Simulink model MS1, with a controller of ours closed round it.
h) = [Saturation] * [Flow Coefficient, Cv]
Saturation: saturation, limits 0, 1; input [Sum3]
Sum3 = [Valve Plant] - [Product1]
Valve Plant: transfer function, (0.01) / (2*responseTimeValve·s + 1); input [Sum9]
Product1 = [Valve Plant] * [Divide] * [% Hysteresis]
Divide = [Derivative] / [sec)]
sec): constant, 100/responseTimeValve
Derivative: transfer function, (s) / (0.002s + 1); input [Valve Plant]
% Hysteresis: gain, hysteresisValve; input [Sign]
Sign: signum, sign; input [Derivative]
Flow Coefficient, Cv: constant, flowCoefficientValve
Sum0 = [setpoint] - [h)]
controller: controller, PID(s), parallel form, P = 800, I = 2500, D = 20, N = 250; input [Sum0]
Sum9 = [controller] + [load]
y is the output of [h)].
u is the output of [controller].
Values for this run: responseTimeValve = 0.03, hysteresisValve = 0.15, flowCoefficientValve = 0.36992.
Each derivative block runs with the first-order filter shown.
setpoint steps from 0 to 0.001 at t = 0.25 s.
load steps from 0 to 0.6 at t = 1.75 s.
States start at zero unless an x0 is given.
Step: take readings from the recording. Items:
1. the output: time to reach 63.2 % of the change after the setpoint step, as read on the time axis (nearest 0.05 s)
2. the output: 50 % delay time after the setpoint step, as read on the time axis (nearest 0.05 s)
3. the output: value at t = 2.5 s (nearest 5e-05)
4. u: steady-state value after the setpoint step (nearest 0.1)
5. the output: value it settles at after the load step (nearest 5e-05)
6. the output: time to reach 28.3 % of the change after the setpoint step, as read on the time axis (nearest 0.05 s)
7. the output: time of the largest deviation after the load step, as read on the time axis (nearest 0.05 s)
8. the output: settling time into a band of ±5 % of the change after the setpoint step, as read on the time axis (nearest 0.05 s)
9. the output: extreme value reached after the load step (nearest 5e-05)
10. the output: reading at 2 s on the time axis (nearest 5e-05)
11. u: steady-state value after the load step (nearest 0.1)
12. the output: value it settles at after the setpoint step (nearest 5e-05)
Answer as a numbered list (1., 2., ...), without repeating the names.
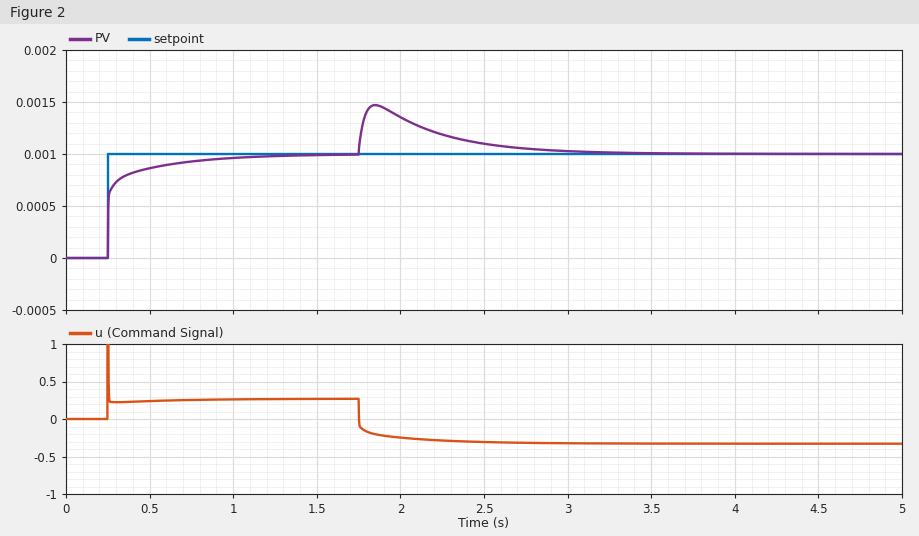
1. 0.25 s
2. 0.25 s
3. 0.00110
4. 0.3
5. 0.00100
6. 0.25 s
7. 1.85 s
8. 0.90 s
9. 0.00145
10. 0.00135
11. -0.3
12. 0.00100
